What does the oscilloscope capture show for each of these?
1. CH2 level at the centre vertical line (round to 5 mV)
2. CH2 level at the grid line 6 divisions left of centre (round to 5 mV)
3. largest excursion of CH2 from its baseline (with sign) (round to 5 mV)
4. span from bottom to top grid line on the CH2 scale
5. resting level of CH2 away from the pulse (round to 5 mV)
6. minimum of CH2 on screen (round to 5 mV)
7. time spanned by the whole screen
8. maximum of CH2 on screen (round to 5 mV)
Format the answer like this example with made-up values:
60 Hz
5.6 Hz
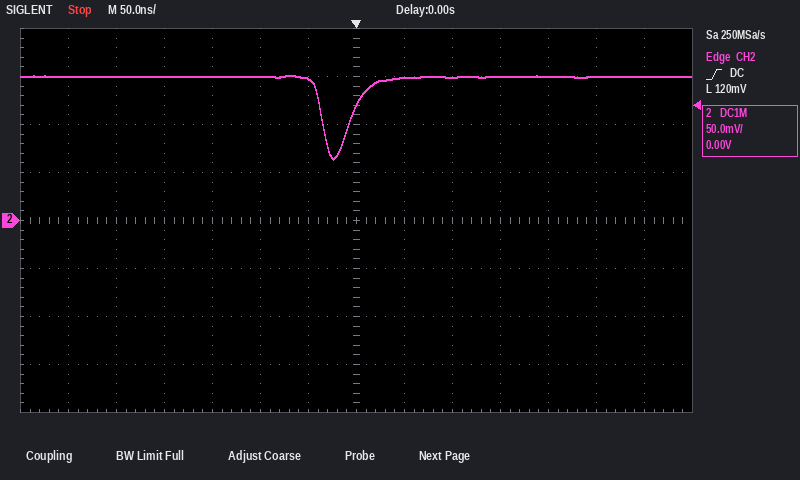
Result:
120 mV
150 mV
-85 mV
400 mV
150 mV
65 mV
700 ns
150 mV
